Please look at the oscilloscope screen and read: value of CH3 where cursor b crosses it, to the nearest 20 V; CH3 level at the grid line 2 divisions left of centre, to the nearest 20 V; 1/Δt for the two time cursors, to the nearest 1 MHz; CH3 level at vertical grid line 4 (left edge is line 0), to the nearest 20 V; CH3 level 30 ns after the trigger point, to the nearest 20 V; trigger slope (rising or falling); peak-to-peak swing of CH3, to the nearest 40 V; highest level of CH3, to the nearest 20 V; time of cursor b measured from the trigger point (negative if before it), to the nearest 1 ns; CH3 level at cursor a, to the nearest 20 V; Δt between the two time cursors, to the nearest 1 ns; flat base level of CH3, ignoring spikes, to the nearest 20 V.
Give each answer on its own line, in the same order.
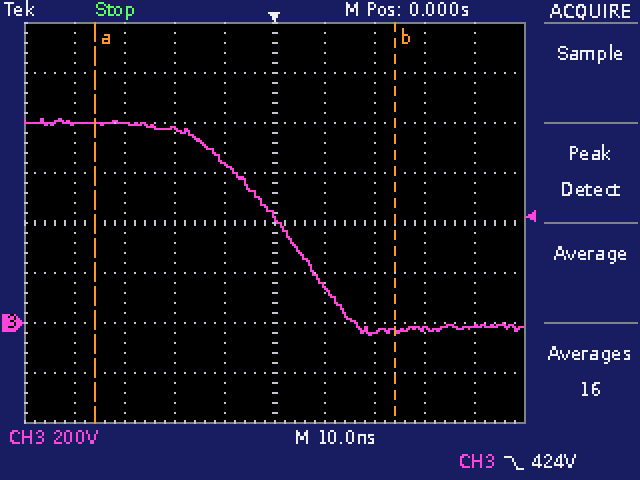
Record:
-40 V
780 V
17 MHz
640 V
-20 V
falling
880 V
820 V
+24 ns
800 V
60 ns
-20 V
